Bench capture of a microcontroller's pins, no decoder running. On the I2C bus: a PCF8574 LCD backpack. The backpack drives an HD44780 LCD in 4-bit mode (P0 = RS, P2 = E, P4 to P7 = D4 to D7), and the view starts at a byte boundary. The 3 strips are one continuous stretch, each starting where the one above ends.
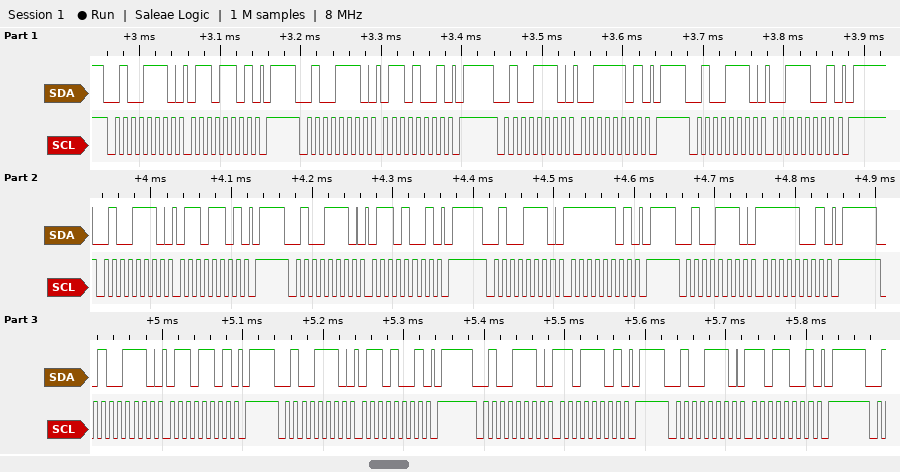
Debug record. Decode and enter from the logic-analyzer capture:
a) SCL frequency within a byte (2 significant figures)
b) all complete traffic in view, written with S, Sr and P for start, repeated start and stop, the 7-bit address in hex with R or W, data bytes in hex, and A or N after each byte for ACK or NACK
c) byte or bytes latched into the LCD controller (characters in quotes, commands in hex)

100 kHz
S 27W A 6D A P S 27W A 69 A P S 27W A 3D A P S 27W A 39 A P S 27W A 6D A P S 27W A 69 A P S 27W A FD A P S 27W A F9 A P S 27W A 6D A P S 27W A 69 A P S 27W A DD A P S 27W A D9 A P
'c' 'o' 'm'
